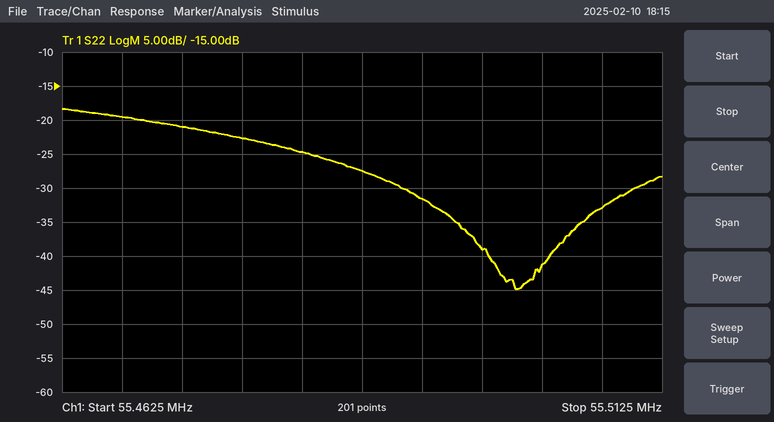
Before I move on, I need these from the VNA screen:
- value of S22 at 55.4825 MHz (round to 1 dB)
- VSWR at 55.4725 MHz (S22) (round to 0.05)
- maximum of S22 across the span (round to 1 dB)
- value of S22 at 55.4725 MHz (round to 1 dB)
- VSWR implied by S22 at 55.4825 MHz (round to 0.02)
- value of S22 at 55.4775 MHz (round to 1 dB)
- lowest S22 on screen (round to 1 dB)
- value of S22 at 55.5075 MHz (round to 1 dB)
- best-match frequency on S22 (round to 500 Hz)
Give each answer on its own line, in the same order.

-25 dB
1.20
-18 dB
-21 dB
1.12
-23 dB
-45 dB
-33 dB
55.5005 MHz
